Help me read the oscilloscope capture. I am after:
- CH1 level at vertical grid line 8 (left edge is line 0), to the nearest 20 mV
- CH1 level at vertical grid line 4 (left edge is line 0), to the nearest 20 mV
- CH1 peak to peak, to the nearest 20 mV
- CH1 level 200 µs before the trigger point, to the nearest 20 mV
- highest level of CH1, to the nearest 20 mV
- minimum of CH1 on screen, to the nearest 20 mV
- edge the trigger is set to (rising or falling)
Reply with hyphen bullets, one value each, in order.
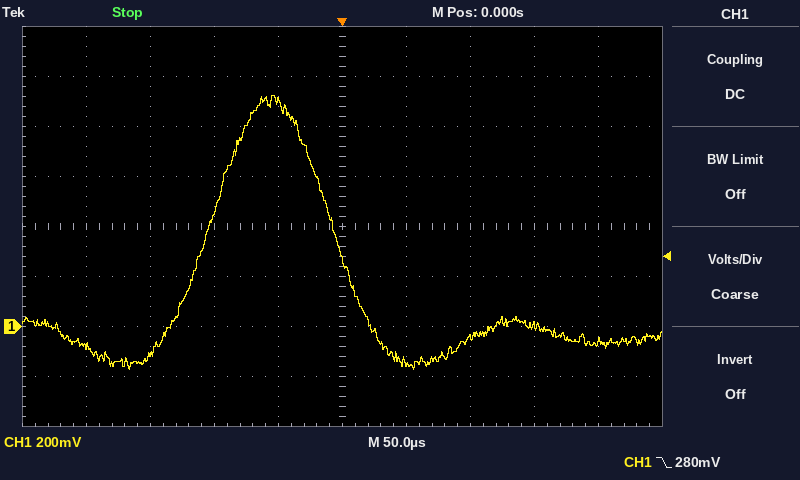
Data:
- 0 mV
- 900 mV
- 1.10 V
- -80 mV
- 920 mV
- -180 mV
- falling
